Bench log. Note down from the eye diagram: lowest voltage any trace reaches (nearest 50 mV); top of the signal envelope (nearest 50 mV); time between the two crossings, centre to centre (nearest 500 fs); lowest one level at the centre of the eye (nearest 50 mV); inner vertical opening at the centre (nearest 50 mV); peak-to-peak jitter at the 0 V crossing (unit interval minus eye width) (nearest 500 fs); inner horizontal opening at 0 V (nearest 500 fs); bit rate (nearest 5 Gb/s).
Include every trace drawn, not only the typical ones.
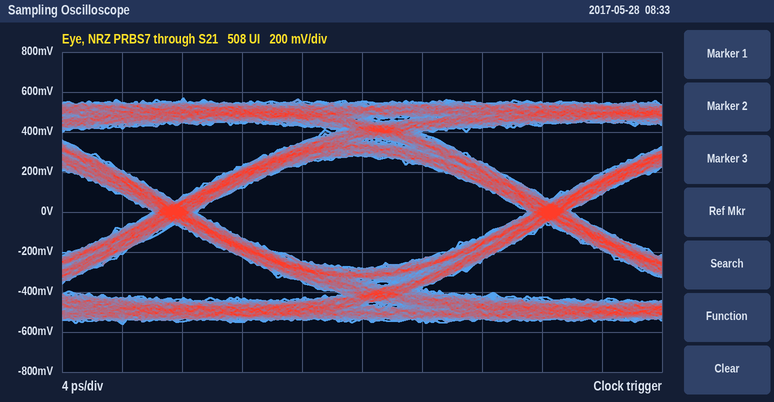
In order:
-550 mV
550 mV
25.0 ps
300 mV
550 mV
3.0 ps
22.0 ps
40 Gb/s
